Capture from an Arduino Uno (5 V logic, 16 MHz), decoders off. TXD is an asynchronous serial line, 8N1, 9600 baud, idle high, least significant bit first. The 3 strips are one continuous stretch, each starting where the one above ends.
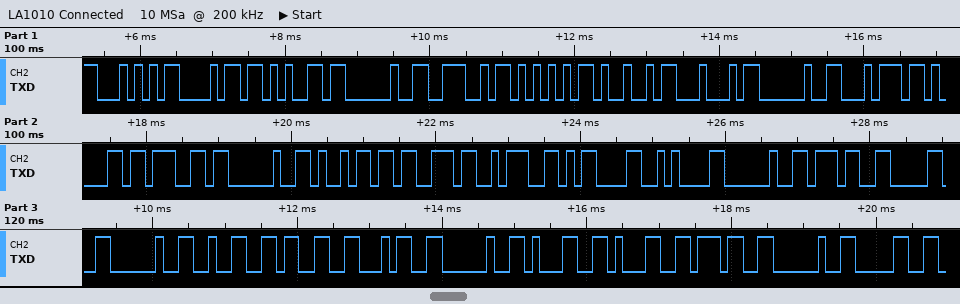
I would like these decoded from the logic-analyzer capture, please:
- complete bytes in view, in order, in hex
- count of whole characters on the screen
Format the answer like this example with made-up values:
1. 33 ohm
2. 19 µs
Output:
1. 54 68 65 20 4E 55 49 44 20 74 61 67 20 69 73 3A 0D 0A 20 37 30 20 32 33 34 20 31 31 37 20 30
2. 31
